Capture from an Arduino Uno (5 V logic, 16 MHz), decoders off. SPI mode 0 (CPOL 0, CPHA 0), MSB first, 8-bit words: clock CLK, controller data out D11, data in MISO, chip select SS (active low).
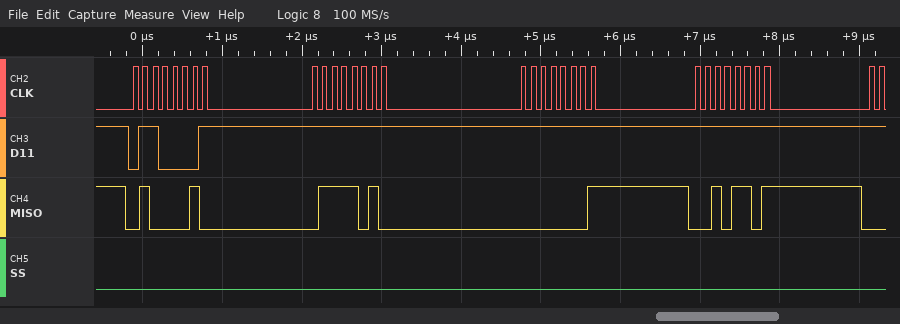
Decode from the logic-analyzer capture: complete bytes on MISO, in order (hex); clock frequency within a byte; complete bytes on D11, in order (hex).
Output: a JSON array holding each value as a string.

["42 7A 01 2D", "8 MHz", "61 FF FF FF"]
